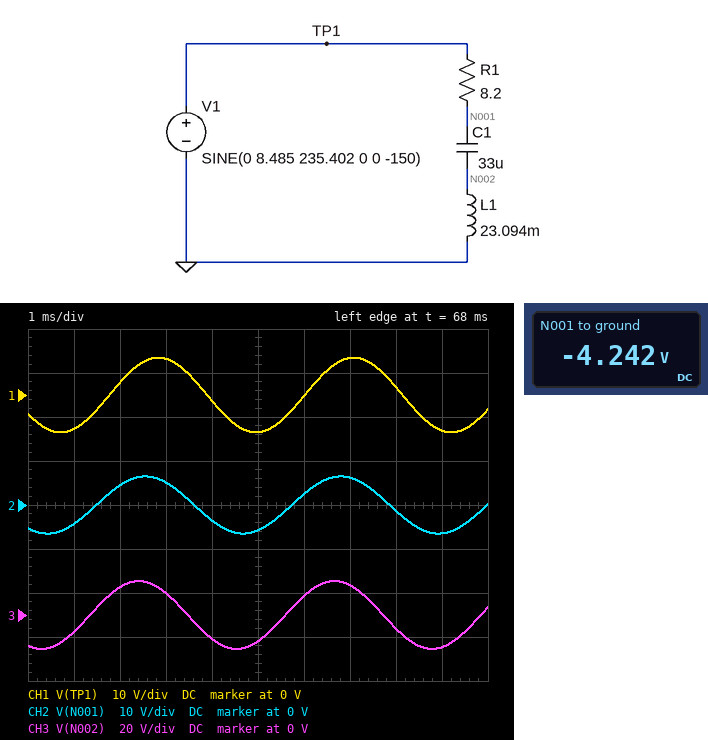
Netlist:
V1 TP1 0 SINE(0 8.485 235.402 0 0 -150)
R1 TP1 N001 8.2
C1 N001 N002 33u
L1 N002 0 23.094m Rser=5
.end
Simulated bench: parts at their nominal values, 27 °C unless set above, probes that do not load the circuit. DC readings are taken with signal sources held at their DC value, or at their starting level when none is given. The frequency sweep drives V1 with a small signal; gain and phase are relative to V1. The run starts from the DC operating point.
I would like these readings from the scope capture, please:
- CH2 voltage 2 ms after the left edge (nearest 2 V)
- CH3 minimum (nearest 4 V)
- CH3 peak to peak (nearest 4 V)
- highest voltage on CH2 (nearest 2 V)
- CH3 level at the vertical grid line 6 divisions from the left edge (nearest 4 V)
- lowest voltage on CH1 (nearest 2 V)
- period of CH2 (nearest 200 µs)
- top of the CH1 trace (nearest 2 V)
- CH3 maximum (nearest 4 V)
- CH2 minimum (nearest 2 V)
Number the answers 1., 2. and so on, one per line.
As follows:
1. 4 V
2. -16 V
3. 32 V
4. 6 V
5. 8 V
6. -8 V
7. 4.2 ms
8. 8 V
9. 16 V
10. -6 V
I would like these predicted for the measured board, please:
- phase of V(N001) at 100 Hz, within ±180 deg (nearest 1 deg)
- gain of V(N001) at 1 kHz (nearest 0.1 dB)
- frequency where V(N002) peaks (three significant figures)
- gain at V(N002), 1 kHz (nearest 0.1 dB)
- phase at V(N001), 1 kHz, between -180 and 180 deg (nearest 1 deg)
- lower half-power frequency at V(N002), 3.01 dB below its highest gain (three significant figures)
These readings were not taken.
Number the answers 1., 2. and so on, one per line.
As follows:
1. -13 deg
2. 0 dB
3. 194 Hz
4. 0.3 dB
5. 3 deg
6. 156 Hz
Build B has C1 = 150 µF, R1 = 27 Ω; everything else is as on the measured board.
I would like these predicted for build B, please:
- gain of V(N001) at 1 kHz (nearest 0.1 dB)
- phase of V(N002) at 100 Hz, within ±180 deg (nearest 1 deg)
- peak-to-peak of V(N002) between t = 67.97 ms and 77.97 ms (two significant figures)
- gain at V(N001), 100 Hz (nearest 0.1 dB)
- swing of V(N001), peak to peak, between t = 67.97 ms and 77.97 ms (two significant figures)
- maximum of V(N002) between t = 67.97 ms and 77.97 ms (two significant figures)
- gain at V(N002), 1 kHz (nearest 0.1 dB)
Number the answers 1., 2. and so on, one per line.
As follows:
1. -0.2 dB
2. 64 deg
3. 13 V
4. -14.1 dB
5. 12 V
6. 6.7 V
7. -0.1 dB
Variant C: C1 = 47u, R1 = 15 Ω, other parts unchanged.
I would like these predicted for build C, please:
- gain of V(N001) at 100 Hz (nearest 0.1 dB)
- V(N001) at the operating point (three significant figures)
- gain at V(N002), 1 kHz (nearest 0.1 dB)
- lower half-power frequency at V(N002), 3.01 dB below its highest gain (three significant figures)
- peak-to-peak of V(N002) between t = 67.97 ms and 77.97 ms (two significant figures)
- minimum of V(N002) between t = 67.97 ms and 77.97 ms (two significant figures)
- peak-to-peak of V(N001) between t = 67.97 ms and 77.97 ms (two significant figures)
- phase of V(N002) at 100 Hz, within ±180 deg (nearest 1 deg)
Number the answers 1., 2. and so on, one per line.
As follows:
1. -2.9 dB
2. -4.24 V
3. 0.1 dB
4. 128 Hz
5. 21 V
6. -10 V
7. 12 V
8. 115 deg
